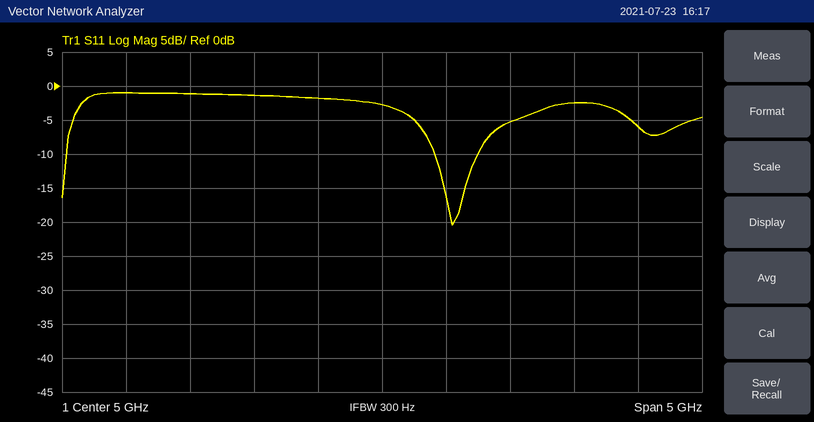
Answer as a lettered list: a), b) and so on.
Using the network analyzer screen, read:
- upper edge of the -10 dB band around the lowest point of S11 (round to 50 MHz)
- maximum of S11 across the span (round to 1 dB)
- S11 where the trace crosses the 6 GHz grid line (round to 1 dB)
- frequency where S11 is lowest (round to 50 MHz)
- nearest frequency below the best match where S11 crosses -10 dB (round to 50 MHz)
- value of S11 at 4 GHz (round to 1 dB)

a) 5.75 GHz
b) -1 dB
c) -5 dB
d) 5.55 GHz
e) 5.40 GHz
f) -1 dB
